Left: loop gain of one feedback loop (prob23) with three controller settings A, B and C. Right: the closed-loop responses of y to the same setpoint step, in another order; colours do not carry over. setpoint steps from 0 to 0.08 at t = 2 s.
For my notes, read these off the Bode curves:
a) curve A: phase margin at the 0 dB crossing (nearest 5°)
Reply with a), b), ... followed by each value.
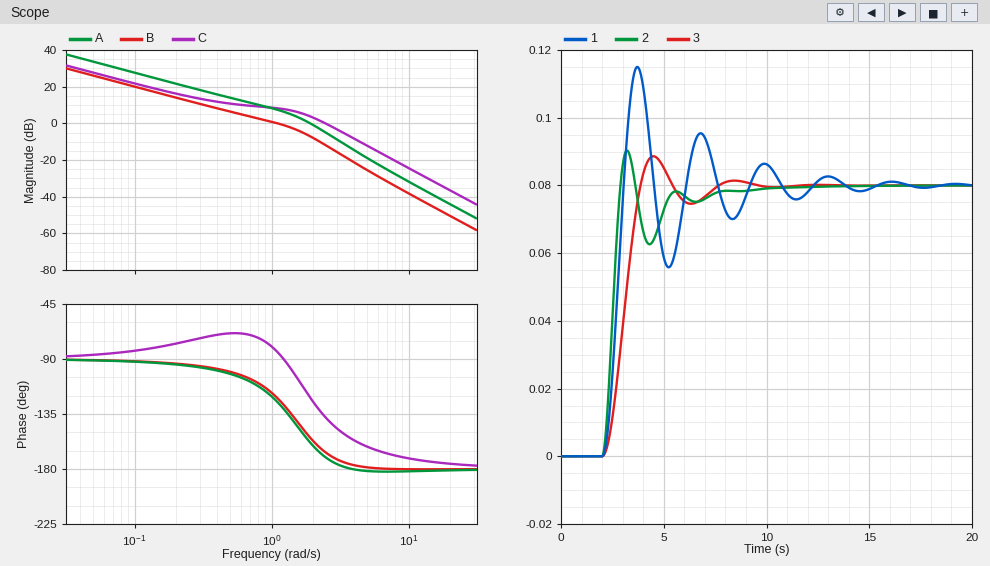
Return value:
a) 20°
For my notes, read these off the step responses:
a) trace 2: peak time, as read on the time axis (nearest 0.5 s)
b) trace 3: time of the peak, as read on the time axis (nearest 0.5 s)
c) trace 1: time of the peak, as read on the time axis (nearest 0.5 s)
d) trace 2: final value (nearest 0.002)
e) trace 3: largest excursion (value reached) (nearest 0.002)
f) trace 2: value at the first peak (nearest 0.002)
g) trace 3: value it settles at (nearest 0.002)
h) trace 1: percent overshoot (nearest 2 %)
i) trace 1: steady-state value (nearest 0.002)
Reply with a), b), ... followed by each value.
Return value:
a) 3.0 s
b) 4.5 s
c) 3.5 s
d) 0.080
e) 0.088
f) 0.090
g) 0.080
h) 44 %
i) 0.080
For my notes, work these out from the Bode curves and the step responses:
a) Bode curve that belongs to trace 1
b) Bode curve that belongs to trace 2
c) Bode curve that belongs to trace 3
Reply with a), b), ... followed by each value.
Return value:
a) A
b) C
c) B
